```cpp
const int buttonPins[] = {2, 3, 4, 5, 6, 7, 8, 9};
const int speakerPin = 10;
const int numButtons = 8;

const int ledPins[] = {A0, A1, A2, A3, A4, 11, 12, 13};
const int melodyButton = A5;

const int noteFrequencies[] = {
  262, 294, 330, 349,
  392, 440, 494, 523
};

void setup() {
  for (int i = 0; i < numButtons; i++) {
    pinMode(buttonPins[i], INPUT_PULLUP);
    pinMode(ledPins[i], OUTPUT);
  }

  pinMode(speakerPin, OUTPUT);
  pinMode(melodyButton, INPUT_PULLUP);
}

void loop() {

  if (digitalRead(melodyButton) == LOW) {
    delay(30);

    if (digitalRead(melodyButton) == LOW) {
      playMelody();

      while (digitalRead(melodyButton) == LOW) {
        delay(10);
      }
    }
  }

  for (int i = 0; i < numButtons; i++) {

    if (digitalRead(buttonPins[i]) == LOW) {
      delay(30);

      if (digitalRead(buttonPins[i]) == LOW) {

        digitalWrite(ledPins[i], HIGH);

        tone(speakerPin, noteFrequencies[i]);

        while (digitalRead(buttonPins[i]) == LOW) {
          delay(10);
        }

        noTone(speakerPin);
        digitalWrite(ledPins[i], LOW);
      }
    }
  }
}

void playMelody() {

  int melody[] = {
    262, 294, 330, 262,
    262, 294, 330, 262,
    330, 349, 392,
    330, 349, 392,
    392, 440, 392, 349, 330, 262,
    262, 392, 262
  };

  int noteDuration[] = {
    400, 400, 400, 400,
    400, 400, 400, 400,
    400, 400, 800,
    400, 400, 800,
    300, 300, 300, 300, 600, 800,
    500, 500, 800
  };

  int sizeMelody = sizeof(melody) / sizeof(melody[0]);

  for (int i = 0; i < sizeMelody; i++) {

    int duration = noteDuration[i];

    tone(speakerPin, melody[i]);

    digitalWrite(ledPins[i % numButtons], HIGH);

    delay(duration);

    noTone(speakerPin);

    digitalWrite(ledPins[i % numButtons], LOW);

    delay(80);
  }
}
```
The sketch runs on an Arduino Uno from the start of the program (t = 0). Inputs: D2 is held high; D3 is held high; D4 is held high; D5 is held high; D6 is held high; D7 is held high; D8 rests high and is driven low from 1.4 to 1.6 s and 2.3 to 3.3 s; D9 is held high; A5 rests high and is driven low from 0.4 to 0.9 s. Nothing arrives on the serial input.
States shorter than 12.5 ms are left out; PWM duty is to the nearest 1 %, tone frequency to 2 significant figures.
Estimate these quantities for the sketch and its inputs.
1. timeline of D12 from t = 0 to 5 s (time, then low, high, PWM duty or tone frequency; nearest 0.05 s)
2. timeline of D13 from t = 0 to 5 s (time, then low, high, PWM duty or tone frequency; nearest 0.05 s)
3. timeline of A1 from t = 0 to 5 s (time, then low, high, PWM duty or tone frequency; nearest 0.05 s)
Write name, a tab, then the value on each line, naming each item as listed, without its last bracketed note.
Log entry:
timeline of D12 from t = 0 to 5 s	0 s low; 3.3 s high; 3.7 s low
timeline of D13 from t = 0 to 5 s	0 s low; 3.8 s high; 4.2 s low
timeline of A1 from t = 0 to 5 s	0 s low; 0.9 s high; 1.3 s low; 4.75 s high
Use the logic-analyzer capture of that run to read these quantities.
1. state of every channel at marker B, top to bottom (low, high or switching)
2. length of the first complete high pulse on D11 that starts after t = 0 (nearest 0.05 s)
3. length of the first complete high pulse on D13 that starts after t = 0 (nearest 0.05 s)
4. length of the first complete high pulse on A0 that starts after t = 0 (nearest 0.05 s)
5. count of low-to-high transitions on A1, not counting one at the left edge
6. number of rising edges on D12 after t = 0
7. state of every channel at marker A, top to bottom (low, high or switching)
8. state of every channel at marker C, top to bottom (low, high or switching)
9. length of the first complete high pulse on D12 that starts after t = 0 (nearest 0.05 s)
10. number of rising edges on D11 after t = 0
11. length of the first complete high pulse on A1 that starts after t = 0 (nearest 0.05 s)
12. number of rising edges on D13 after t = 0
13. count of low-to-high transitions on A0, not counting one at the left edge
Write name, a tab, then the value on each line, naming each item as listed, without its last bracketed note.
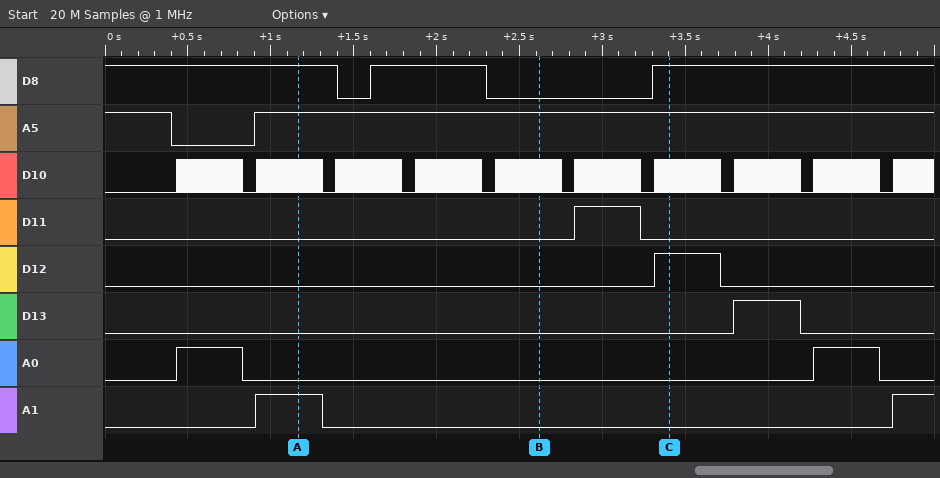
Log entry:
state of every channel at marker B, top to bottom	D8 low, A5 high, D10 switching, D11 low, D12 low, D13 low, A0 low, A1 low
length of the first complete high pulse on D11 that starts after t = 0	0.40 s
length of the first complete high pulse on D13 that starts after t = 0	0.40 s
length of the first complete high pulse on A0 that starts after t = 0	0.40 s
count of low-to-high transitions on A1, not counting one at the left edge	2
number of rising edges on D12 after t = 0	1
state of every channel at marker A, top to bottom	D8 high, A5 high, D10 switching, D11 low, D12 low, D13 low, A0 low, A1 high
state of every channel at marker C, top to bottom	D8 high, A5 high, D10 switching, D11 low, D12 high, D13 low, A0 low, A1 low
length of the first complete high pulse on D12 that starts after t = 0	0.40 s
number of rising edges on D11 after t = 0	1
length of the first complete high pulse on A1 that starts after t = 0	0.40 s
number of rising edges on D13 after t = 0	1
count of low-to-high transitions on A0, not counting one at the left edge	2
